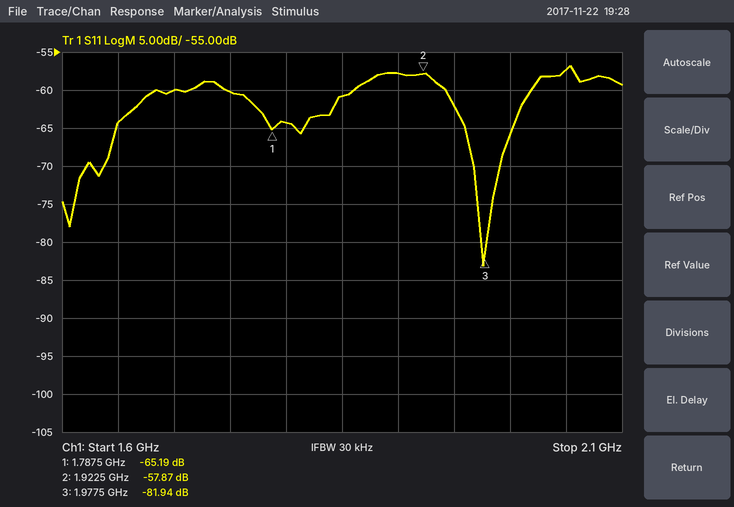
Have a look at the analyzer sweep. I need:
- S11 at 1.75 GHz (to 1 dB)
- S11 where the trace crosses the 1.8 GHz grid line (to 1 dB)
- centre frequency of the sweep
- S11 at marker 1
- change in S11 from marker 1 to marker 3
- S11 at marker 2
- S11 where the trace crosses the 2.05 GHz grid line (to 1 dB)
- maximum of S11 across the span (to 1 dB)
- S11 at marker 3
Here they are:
-60 dB
-64 dB
1.85 GHz
-65.19 dB
-16.75 dB
-57.87 dB
-57 dB
-57 dB
-81.94 dB
